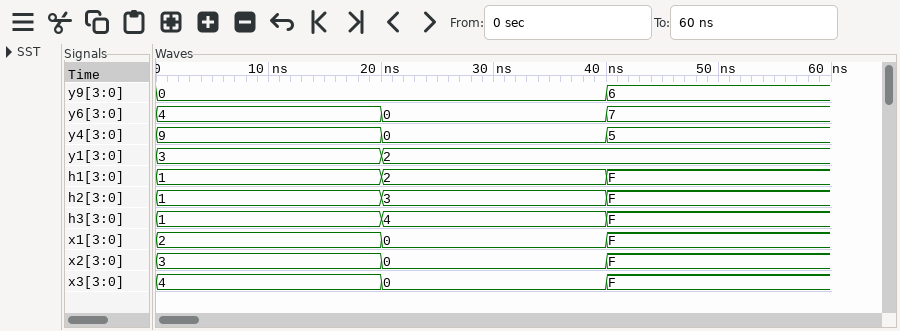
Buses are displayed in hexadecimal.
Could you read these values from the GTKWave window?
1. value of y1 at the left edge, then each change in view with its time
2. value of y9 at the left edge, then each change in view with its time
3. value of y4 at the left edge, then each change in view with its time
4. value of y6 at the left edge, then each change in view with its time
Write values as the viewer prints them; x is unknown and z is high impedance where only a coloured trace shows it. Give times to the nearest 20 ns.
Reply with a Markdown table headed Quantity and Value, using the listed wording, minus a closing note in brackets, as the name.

| Quantity | Value |
|---|---|
| value of y1 at the left edge, then each change in view with its time | 3, 2 at 20 ns |
| value of y9 at the left edge, then each change in view with its time | 0, 6 at 40 ns |
| value of y4 at the left edge, then each change in view with its time | 9, 0 at 20 ns, 5 at 40 ns |
| value of y6 at the left edge, then each change in view with its time | 4, 0 at 20 ns, 7 at 40 ns |
